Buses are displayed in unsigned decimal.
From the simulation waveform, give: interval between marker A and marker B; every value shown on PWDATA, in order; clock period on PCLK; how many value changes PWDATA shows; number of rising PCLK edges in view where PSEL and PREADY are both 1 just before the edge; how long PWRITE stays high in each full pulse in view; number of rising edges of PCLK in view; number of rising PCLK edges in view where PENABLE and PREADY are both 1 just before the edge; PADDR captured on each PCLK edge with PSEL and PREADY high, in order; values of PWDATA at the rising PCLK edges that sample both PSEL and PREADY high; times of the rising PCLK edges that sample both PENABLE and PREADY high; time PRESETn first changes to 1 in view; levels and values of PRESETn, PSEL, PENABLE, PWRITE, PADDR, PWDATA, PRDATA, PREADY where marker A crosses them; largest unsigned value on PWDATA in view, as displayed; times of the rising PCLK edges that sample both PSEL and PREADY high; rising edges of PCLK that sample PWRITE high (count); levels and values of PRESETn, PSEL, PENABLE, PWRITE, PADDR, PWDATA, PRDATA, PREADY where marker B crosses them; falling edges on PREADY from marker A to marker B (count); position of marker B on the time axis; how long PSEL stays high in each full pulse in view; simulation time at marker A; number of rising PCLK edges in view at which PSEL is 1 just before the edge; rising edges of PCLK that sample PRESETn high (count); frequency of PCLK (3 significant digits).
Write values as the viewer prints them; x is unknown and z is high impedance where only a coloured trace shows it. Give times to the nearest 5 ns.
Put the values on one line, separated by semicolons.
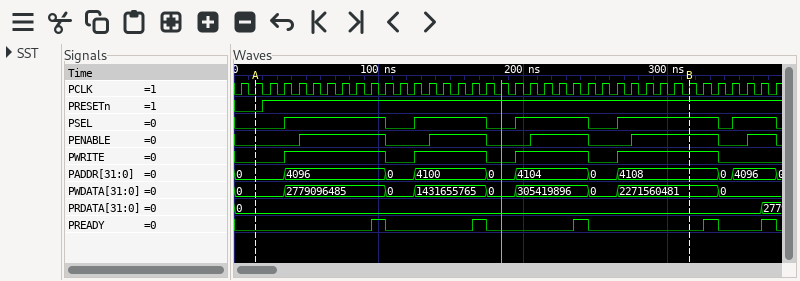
300 ns; 0, 2779096485, 0, 1431655765, 0, 305419896, 0, 2271560481, 0; 10 ns; 8; 5; 70 ns, 50 ns, 50 ns, 70 ns; 38; 5; 4096, 4100, 4104, 4108, 4096; 2779096485, 1431655765, 305419896, 2271560481, 0; 105 ns, 175 ns, 245 ns, 335 ns, 375 ns; 20 ns; PRESETn=0, PSEL=0, PENABLE=0, PWRITE=0, PADDR=0, PWDATA=0, PRDATA=0, PREADY=0; 2779096485; 105 ns, 175 ns, 245 ns, 335 ns, 375 ns; 24; PRESETn=1, PSEL=1, PENABLE=1, PWRITE=1, PADDR=4108, PWDATA=2271560481, PRDATA=0, PREADY=0; 3; 315 ns; 70 ns, 50 ns, 50 ns, 70 ns, 30 ns; 15 ns; 27; 36; 100 MHz
